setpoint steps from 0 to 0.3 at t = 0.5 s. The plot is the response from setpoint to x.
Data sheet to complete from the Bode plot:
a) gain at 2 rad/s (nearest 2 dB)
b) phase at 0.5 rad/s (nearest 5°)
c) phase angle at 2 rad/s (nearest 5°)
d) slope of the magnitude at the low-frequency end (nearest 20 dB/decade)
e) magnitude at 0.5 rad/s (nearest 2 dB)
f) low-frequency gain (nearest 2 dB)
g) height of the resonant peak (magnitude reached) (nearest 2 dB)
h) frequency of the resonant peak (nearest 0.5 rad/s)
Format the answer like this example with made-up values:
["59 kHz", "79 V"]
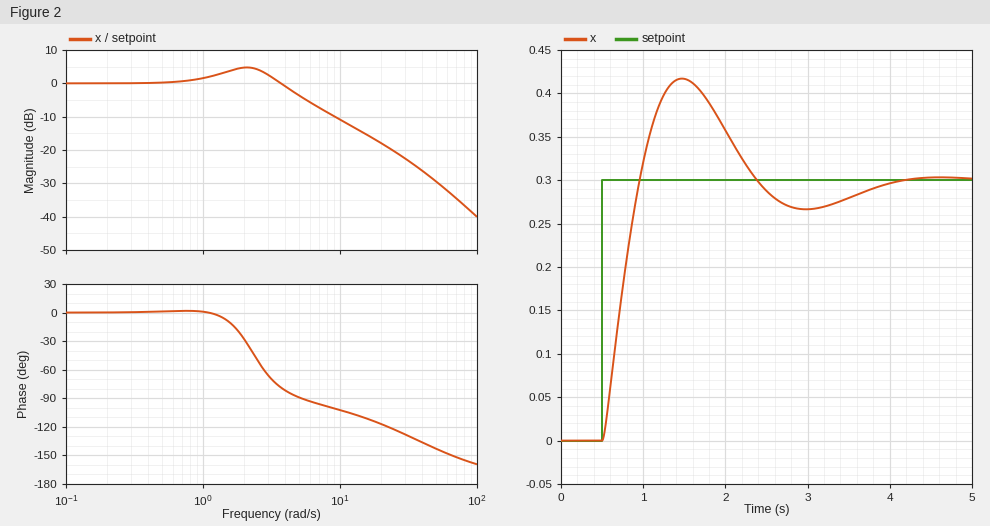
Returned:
["4 dB", "0°", "-30°", "0 dB/decade", "0 dB", "0 dB", "4 dB", "2.0 rad/s"]
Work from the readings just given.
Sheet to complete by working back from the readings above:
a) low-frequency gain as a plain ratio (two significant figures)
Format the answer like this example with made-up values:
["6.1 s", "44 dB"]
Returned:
["1.0"]
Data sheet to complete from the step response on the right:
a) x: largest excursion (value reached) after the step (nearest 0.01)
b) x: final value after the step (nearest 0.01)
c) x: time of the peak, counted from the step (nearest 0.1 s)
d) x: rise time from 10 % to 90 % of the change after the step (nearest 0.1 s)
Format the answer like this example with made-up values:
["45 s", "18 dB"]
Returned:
["0.42", "0.30", "1.0 s", "0.3 s"]
